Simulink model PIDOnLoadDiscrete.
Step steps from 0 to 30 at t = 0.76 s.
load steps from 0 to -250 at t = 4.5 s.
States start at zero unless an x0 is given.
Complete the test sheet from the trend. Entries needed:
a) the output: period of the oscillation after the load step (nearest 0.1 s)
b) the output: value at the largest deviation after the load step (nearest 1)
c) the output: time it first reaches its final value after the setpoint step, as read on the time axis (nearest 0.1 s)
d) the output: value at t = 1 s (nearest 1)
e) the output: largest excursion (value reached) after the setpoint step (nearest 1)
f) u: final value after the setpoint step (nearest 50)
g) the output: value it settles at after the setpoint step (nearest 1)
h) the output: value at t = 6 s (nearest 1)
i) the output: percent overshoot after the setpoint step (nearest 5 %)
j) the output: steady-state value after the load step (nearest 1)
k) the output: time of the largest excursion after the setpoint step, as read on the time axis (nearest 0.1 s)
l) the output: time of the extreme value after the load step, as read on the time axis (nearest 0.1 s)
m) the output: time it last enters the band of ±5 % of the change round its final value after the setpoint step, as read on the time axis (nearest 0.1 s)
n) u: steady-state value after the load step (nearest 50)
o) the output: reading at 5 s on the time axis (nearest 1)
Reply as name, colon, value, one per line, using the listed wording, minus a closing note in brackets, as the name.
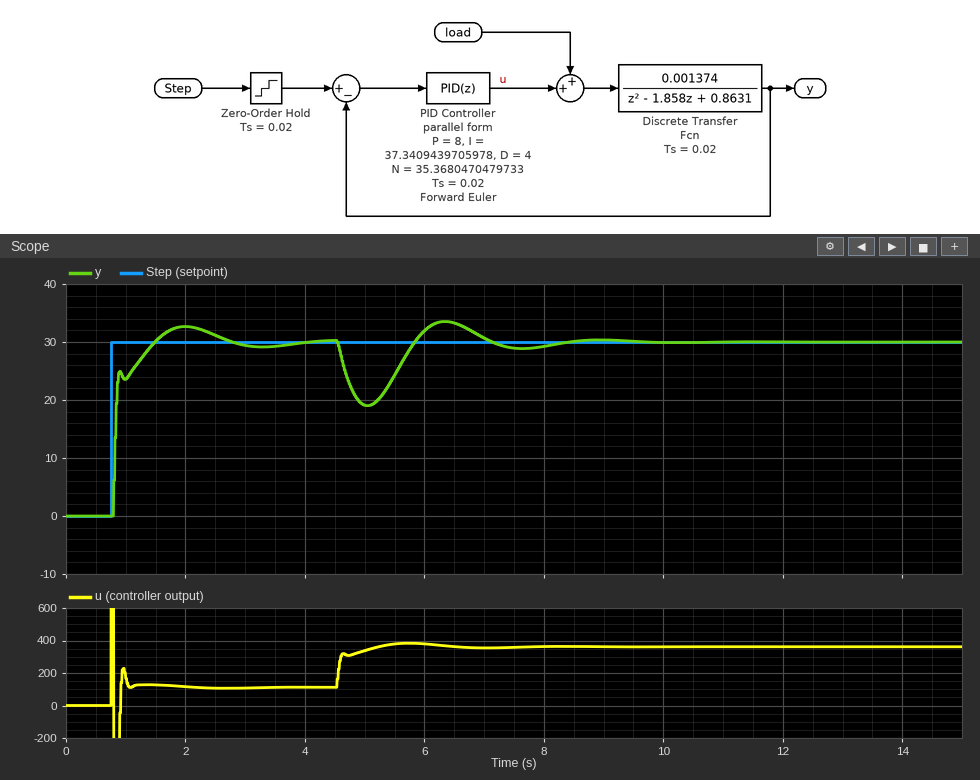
the output: period of the oscillation after the load step: 2.6 s
the output: value at the largest deviation after the load step: 19
the output: time it first reaches its final value after the setpoint step, as read on the time axis: 1.5 s
the output: value at t = 1 s: 24
the output: largest excursion (value reached) after the setpoint step: 33
u: final value after the setpoint step: 100
the output: value it settles at after the setpoint step: 30
the output: value at t = 6 s: 32
the output: percent overshoot after the setpoint step: 10 %
the output: steady-state value after the load step: 30
the output: time of the largest excursion after the setpoint step, as read on the time axis: 2.0 s
the output: time of the extreme value after the load step, as read on the time axis: 5.0 s
the output: time it last enters the band of ±5 % of the change round its final value after the setpoint step, as read on the time axis: 2.4 s
u: steady-state value after the load step: 350
the output: reading at 5 s on the time axis: 19
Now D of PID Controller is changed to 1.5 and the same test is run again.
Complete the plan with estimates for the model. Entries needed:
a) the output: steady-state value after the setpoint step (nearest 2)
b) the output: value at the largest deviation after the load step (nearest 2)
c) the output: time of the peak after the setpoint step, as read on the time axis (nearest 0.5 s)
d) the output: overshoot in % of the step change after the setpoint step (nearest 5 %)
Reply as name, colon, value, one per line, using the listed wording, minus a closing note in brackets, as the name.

the output: steady-state value after the setpoint step: 30
the output: value at the largest deviation after the load step: 16
the output: time of the peak after the setpoint step, as read on the time axis: 1.5 s
the output: overshoot in % of the step change after the setpoint step: 15 %
